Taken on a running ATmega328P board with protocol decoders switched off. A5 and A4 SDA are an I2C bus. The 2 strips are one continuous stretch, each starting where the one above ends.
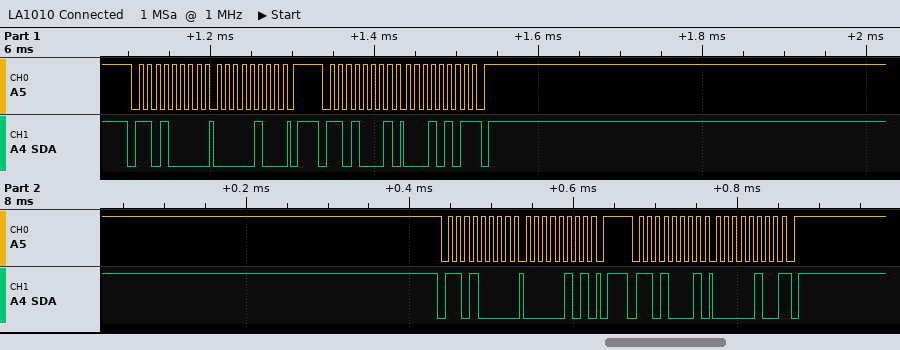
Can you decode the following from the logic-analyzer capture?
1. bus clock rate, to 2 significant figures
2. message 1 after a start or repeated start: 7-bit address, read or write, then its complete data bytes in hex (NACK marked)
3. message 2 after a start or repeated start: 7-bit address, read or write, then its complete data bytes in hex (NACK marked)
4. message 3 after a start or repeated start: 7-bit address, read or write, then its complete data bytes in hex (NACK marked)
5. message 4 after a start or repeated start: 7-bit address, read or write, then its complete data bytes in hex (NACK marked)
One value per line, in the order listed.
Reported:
100 kHz
0x68 write: 04
0x68 read: 15 NACK
0x68 write: 05
0x68 read: 04 NACK
